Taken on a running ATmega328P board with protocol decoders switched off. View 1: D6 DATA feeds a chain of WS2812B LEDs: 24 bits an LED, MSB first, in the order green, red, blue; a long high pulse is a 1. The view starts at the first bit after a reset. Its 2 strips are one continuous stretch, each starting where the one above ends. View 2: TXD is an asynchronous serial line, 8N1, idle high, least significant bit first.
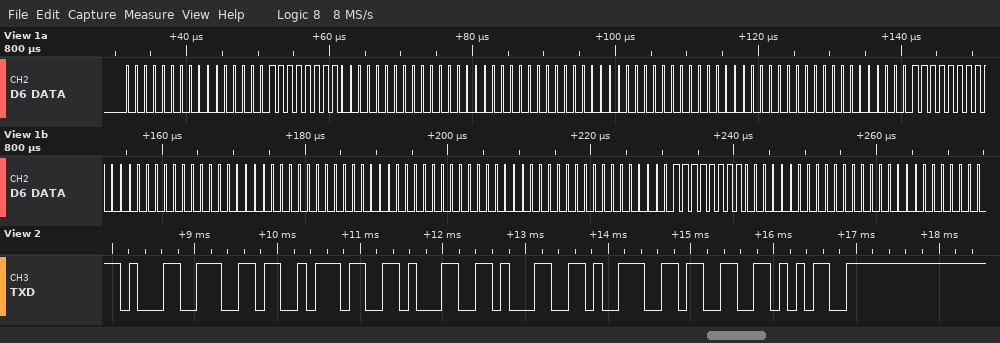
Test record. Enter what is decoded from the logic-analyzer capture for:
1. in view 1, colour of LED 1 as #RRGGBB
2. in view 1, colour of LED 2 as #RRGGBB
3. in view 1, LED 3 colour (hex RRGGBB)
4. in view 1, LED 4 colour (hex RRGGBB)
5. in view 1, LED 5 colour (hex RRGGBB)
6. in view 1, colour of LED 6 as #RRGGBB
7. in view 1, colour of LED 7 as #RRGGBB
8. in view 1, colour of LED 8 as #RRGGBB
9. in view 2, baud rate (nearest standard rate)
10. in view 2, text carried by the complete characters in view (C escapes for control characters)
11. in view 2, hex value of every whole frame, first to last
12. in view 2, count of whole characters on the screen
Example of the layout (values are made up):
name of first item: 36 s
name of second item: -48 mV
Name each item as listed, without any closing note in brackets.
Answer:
in view 1, colour of LED 1 as #RRGGBB: #0000FF
in view 1, colour of LED 2 as #RRGGBB: #000000
in view 1, LED 3 colour: #000000
in view 1, LED 4 colour: #0000FF
in view 1, LED 5 colour: #000000
in view 1, colour of LED 6 as #RRGGBB: #000000
in view 1, colour of LED 7 as #RRGGBB: #0000FF
in view 1, colour of LED 8 as #RRGGBB: #000000
in view 2, baud rate: 9600 baud
in view 2, text carried by the complete characters in view: "16711935"
in view 2, hex value of every whole frame, first to last: 31 36 37 31 31 39 33 35
in view 2, count of whole characters on the screen: 8
